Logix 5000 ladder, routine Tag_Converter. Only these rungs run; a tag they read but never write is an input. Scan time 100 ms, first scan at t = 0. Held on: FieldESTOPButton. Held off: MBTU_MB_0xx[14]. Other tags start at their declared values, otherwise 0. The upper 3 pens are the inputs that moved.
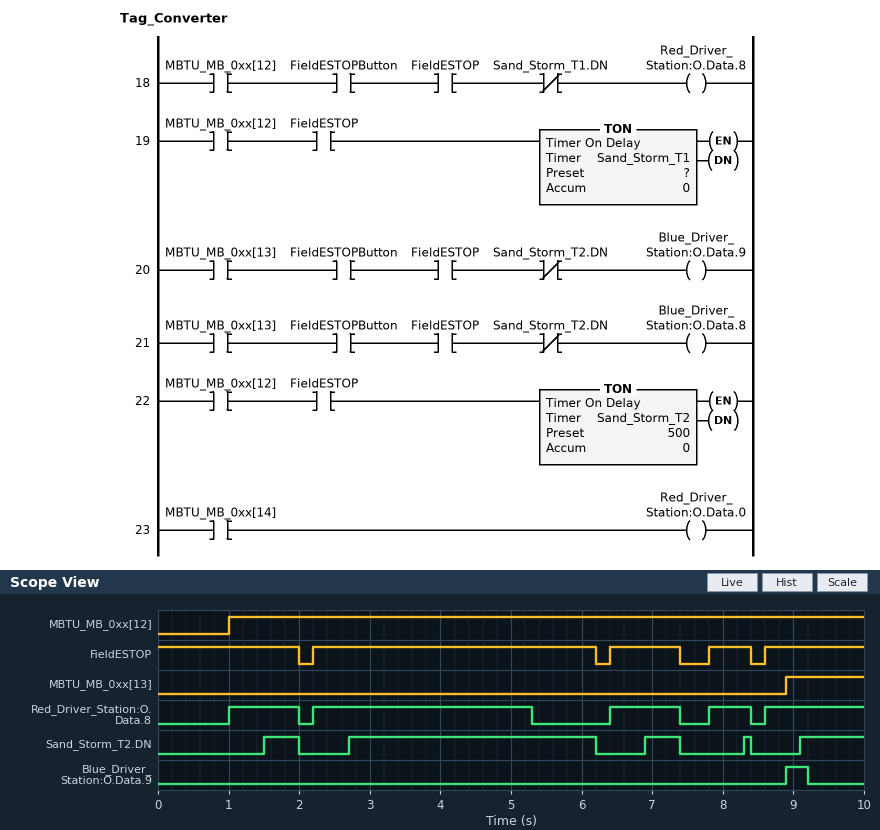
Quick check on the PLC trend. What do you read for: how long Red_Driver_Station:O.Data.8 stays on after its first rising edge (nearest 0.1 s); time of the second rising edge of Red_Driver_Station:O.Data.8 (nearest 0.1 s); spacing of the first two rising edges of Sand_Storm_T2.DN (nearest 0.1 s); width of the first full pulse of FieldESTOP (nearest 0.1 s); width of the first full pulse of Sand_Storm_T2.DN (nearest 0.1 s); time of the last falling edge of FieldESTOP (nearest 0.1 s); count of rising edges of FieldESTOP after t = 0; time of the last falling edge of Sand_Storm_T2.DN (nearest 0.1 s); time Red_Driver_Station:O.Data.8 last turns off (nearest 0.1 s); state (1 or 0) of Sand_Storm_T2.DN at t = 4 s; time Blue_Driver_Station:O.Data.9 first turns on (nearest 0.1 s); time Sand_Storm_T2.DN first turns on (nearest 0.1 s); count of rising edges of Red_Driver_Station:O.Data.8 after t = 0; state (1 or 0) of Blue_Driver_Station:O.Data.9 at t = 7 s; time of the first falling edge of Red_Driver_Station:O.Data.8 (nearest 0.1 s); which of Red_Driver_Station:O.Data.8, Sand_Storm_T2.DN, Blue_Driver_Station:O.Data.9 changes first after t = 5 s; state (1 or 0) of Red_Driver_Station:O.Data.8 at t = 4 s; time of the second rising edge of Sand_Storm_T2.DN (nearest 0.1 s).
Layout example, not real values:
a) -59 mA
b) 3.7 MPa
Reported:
a) 1.0 s
b) 2.2 s
c) 1.2 s
d) 4.0 s
e) 0.5 s
f) 8.4 s
g) 4
h) 8.4 s
i) 8.4 s
j) 1
k) 8.9 s
l) 1.5 s
m) 5
n) 0
o) 2.0 s
p) Red_Driver_Station:O.Data.8
q) 1
r) 2.7 s
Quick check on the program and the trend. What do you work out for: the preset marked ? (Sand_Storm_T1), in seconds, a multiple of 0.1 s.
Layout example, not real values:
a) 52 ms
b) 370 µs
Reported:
a) 3.0 s
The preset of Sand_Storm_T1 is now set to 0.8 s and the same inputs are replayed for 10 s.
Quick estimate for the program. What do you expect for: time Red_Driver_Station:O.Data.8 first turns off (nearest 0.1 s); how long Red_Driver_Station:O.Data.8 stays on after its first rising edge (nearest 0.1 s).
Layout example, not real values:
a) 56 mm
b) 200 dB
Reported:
a) 1.9 s
b) 0.9 s
